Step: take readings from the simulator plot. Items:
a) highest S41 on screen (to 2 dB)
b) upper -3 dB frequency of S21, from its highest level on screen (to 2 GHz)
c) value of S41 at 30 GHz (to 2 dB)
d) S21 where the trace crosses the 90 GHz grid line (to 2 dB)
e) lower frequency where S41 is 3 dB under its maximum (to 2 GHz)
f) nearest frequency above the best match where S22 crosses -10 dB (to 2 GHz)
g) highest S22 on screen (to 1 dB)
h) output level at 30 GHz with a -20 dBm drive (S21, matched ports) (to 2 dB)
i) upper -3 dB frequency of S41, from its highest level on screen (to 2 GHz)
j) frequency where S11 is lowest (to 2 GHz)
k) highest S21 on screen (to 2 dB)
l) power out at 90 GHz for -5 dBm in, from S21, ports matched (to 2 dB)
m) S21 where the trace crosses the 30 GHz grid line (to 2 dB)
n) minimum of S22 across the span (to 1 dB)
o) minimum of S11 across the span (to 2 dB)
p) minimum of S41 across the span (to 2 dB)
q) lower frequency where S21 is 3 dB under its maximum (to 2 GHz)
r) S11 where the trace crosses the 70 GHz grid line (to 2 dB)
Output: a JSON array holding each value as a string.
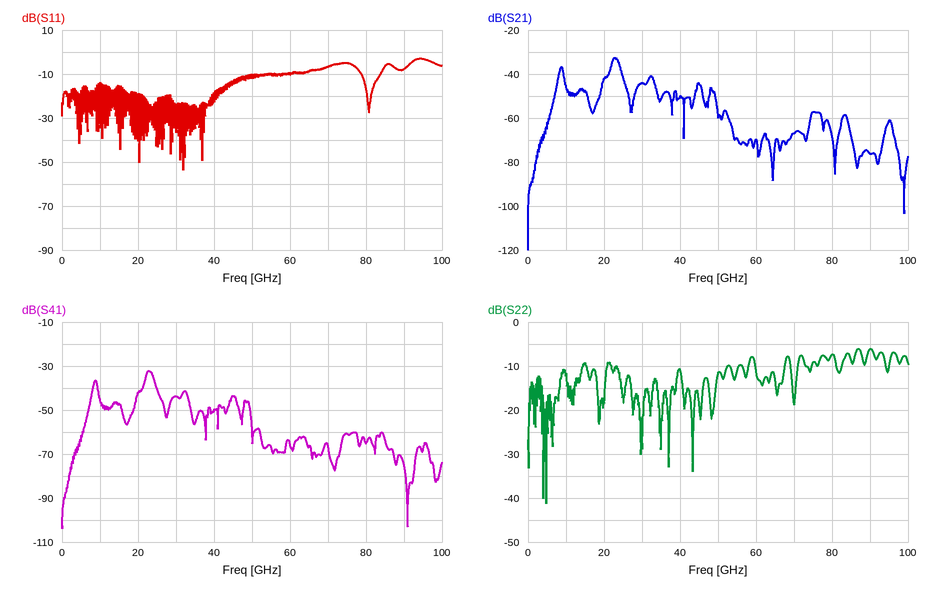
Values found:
["-32 dB", "24 GHz", "-44 dB", "-76 dB", "22 GHz", "14 GHz", "-6 dB", "-64 dBm", "24 GHz", "32 GHz", "-32 dB", "-82 dBm", "-44 dB", "-41 dB", "-54 dB", "-104 dB", "22 GHz", "-6 dB"]
